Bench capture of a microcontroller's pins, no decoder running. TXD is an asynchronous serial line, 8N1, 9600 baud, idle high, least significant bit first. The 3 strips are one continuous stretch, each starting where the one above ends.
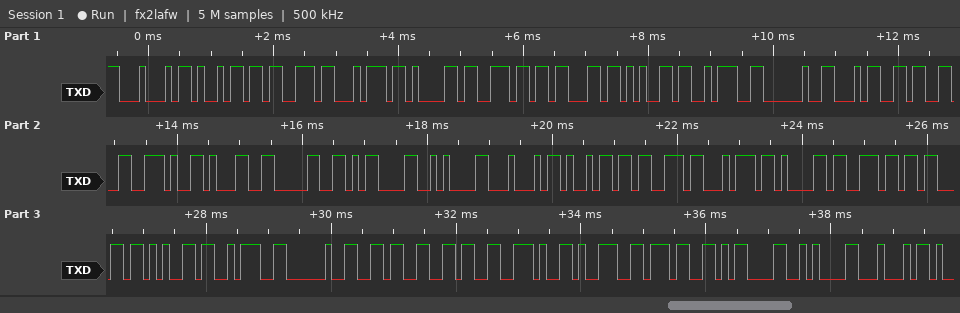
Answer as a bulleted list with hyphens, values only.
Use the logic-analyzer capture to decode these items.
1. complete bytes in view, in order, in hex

- 0x44 0x69 0x73 0x74 0x61 0x6E 0x63 0x65 0x3A 0x20 0x34 0x33 0x2E 0x31 0x30 0x0D 0x0A 0x44 0x69 0x73 0x74 0x61 0x6E 0x63 0x65 0x3A 0x20 0x36 0x36 0x2E 0x39 0x37 0x0D 0x0A 0x44
